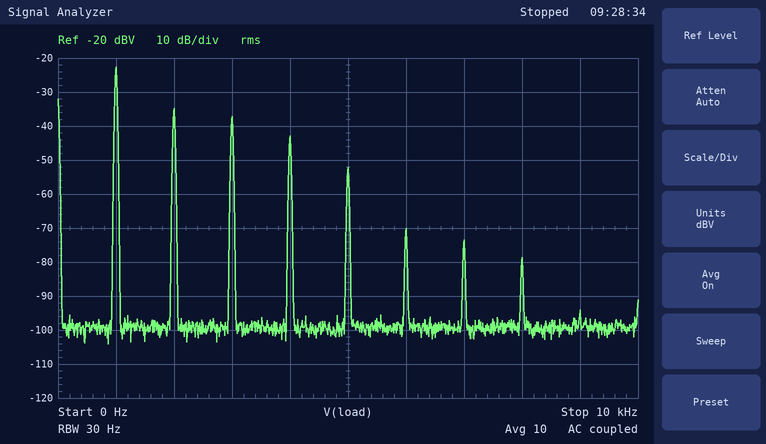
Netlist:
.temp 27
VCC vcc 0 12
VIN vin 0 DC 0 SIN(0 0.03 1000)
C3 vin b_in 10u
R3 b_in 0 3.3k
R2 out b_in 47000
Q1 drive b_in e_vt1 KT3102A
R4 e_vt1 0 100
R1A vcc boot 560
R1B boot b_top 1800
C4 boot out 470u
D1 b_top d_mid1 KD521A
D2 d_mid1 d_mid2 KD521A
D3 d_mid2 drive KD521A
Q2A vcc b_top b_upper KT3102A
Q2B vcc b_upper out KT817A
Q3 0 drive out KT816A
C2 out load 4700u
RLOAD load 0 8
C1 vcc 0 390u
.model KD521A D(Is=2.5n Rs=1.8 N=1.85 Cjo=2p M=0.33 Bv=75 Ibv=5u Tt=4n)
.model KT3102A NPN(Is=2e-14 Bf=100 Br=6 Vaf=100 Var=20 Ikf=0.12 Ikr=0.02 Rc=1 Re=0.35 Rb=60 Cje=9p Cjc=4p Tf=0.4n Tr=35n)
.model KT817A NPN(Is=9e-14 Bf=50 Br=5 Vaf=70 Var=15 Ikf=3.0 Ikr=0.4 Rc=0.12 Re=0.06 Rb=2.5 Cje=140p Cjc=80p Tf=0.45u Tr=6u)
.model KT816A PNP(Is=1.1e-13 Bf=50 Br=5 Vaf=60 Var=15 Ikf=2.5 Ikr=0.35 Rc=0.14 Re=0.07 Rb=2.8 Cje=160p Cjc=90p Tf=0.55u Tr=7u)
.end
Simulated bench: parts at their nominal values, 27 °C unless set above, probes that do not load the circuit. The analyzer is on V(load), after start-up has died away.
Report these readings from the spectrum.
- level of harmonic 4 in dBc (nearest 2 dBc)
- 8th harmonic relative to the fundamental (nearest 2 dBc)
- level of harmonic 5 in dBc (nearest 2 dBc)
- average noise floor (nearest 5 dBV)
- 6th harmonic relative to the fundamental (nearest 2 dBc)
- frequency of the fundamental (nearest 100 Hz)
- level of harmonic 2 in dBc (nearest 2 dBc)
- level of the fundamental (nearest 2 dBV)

-20 dBc
-56 dBc
-30 dBc
-100 dBV
-48 dBc
1.0 kHz
-12 dBc
-22 dBV
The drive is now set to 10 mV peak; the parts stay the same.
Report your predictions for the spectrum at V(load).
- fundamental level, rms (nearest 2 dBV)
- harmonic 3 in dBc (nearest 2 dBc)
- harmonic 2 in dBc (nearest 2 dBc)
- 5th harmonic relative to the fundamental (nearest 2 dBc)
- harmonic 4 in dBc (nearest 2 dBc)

-36 dBV
-24 dBc
-22 dBc
-50 dBc
-34 dBc
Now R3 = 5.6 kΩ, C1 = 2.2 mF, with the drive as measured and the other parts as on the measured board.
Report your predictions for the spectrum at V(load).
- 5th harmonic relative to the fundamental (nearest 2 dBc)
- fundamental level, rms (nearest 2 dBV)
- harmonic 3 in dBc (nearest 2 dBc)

-26 dBc
-18 dBV
-16 dBc
